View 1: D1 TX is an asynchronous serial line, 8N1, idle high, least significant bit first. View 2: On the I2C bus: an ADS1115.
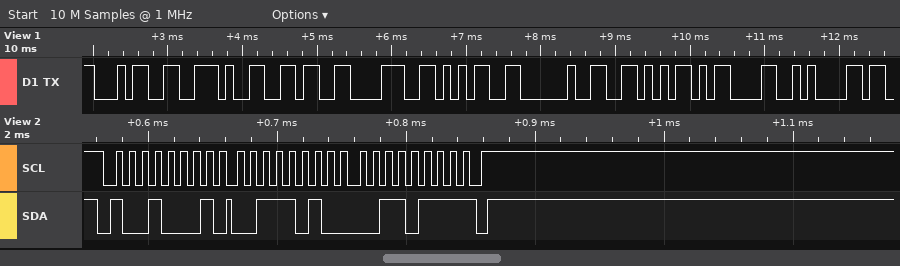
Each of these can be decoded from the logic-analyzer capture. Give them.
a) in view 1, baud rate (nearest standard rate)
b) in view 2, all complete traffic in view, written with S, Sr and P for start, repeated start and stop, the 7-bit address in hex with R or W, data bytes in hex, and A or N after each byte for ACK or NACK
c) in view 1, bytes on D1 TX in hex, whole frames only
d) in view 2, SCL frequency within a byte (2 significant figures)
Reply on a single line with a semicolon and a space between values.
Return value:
9600 baud; S 48R A 3A A 37 N P; 34 2E 36 38 35 20 56 0D 0A; 100 kHz
